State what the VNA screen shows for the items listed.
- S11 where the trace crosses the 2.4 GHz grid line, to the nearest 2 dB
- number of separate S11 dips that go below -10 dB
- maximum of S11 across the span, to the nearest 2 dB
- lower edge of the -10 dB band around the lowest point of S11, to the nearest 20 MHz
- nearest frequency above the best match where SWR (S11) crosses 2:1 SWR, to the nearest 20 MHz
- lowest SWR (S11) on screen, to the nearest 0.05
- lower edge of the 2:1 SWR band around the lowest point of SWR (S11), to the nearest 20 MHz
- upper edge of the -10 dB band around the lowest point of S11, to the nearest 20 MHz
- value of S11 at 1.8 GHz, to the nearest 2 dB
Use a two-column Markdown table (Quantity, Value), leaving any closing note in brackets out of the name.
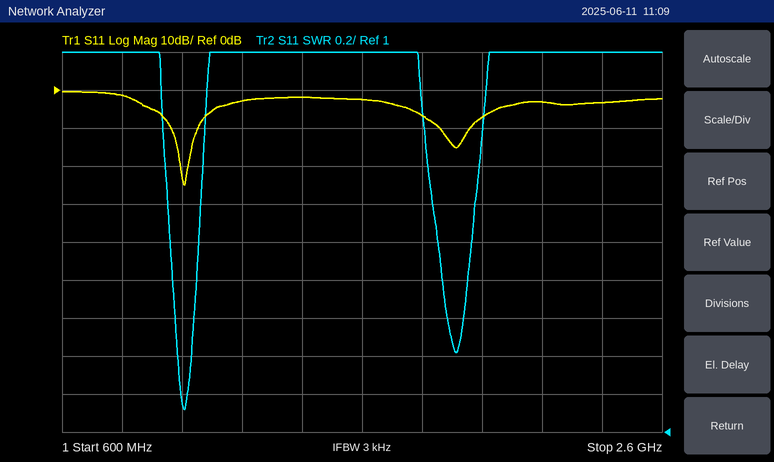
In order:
| Quantity | Value |
|---|---|
| S11 where the trace crosses the 2.4 GHz grid line, to the nearest 2 dB | -4 dB |
| number of separate S11 dips that go below -10 dB | 2 |
| maximum of S11 across the span, to the nearest 2 dB | 0 dB |
| lower edge of the -10 dB band around the lowest point of S11, to the nearest 20 MHz | 960 MHz |
| nearest frequency above the best match where SWR (S11) crosses 2:1 SWR, to the nearest 20 MHz | 1.06 GHz |
| lowest SWR (S11) on screen, to the nearest 0.05 | 1.10 |
| lower edge of the 2:1 SWR band around the lowest point of SWR (S11), to the nearest 20 MHz | 960 MHz |
| upper edge of the -10 dB band around the lowest point of S11, to the nearest 20 MHz | 1.06 GHz |
| value of S11 at 1.8 GHz, to the nearest 2 dB | -6 dB |
